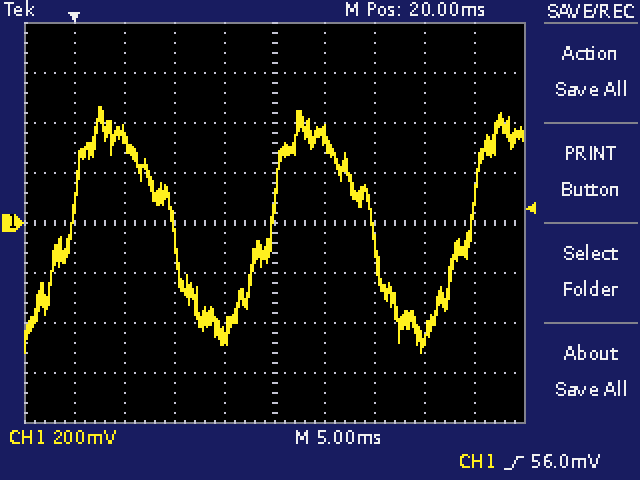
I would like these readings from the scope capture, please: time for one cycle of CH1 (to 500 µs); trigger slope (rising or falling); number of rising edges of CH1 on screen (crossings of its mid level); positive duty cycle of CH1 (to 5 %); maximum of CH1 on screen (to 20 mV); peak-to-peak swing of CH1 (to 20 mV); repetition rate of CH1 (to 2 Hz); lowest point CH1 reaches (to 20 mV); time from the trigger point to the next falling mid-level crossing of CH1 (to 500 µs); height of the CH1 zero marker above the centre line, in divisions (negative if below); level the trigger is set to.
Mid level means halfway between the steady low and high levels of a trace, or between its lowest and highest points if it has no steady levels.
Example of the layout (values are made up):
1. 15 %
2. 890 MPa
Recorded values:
1. 20.0 ms
2. rising
3. 3
4. 50 %
5. 460 mV
6. 980 mV
7. 50 Hz
8. -520 mV
9. 10.0 ms
10. 0.0 div
11. 56.0 mV
